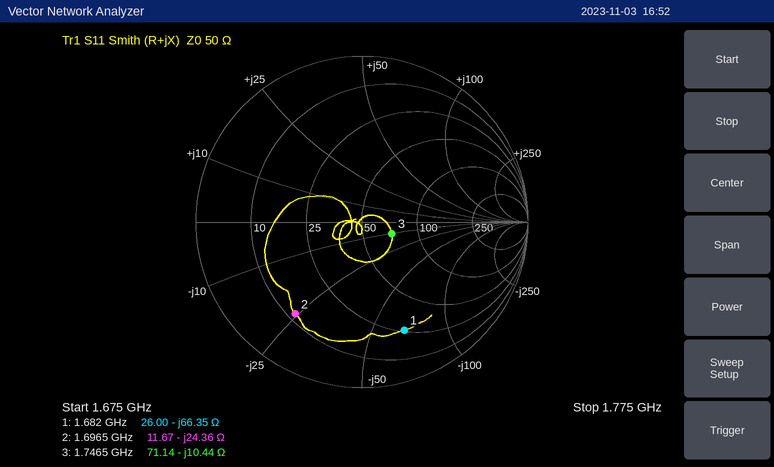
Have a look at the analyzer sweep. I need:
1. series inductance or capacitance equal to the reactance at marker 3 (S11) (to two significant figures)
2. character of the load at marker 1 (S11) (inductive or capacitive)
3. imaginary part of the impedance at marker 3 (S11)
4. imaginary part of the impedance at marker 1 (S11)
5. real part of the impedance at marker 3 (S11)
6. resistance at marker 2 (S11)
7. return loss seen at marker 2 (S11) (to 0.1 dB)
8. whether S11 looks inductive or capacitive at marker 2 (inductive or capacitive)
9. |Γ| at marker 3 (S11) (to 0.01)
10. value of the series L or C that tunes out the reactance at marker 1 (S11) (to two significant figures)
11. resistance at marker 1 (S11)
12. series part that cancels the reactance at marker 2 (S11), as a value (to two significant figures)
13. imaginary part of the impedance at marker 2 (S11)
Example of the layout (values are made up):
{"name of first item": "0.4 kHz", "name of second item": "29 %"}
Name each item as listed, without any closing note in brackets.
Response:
{"series inductance or capacitance equal to the reactance at marker 3 (S11)": "8.7 pF", "character of the load at marker 1 (S11)": "capacitive", "imaginary part of the impedance at marker 3": "-10.44 Ω", "imaginary part of the impedance at marker 1": "-66.35 Ω", "real part of the impedance at marker 3": "71.14 Ω", "resistance at marker 2": "11.67 Ω", "return loss seen at marker 2 (S11)": "3.3 dB", "whether S11 looks inductive or capacitive at marker 2": "capacitive", "|Γ| at marker 3 (S11)": "0.19", "value of the series L or C that tunes out the reactance at marker 1 (S11)": "6.3 nH", "resistance at marker 1": "26.00 Ω", "series part that cancels the reactance at marker 2 (S11), as a value": "2.3 nH", "imaginary part of the impedance at marker 2": "-24.36 Ω"}
